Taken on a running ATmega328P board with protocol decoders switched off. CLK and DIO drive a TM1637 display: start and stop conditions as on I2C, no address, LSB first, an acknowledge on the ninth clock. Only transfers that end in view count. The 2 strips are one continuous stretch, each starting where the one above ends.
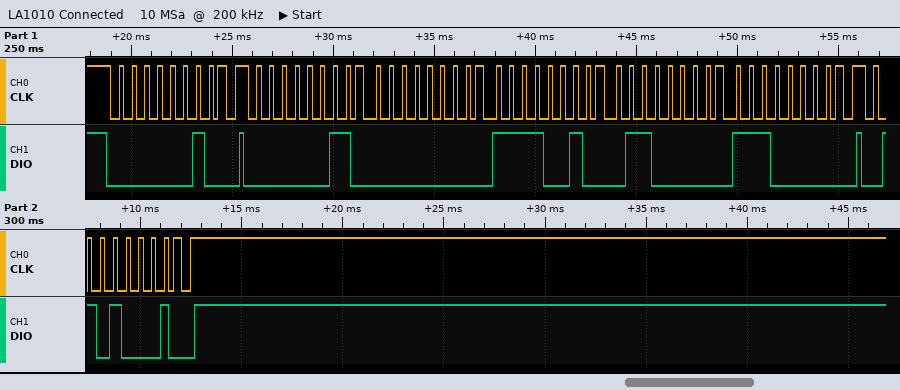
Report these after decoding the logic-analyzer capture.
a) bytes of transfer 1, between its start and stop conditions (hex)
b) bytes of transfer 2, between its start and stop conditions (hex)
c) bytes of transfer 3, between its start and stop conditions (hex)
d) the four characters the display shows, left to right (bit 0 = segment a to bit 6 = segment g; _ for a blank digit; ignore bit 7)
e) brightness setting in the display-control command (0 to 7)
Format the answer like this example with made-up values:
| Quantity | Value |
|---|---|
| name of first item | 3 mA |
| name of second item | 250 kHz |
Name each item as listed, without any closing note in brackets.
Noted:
| Quantity | Value |
|---|---|
| bytes of transfer 1, between its start and stop conditions | 40 |
| bytes of transfer 2, between its start and stop conditions | C0 00 4F 06 07 |
| bytes of transfer 3, between its start and stop conditions | 8A |
| the four characters the display shows, left to right | _317 |
| brightness setting in the display-control command | 2 |
